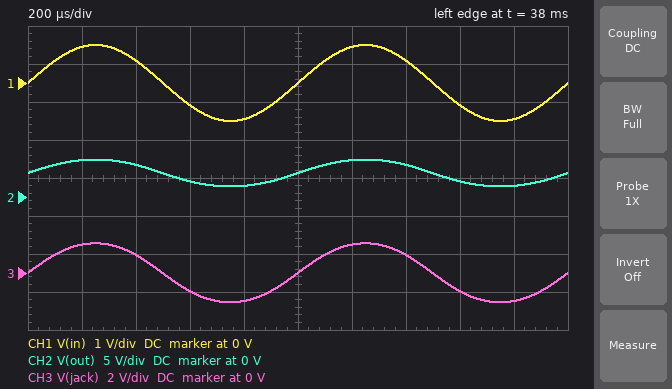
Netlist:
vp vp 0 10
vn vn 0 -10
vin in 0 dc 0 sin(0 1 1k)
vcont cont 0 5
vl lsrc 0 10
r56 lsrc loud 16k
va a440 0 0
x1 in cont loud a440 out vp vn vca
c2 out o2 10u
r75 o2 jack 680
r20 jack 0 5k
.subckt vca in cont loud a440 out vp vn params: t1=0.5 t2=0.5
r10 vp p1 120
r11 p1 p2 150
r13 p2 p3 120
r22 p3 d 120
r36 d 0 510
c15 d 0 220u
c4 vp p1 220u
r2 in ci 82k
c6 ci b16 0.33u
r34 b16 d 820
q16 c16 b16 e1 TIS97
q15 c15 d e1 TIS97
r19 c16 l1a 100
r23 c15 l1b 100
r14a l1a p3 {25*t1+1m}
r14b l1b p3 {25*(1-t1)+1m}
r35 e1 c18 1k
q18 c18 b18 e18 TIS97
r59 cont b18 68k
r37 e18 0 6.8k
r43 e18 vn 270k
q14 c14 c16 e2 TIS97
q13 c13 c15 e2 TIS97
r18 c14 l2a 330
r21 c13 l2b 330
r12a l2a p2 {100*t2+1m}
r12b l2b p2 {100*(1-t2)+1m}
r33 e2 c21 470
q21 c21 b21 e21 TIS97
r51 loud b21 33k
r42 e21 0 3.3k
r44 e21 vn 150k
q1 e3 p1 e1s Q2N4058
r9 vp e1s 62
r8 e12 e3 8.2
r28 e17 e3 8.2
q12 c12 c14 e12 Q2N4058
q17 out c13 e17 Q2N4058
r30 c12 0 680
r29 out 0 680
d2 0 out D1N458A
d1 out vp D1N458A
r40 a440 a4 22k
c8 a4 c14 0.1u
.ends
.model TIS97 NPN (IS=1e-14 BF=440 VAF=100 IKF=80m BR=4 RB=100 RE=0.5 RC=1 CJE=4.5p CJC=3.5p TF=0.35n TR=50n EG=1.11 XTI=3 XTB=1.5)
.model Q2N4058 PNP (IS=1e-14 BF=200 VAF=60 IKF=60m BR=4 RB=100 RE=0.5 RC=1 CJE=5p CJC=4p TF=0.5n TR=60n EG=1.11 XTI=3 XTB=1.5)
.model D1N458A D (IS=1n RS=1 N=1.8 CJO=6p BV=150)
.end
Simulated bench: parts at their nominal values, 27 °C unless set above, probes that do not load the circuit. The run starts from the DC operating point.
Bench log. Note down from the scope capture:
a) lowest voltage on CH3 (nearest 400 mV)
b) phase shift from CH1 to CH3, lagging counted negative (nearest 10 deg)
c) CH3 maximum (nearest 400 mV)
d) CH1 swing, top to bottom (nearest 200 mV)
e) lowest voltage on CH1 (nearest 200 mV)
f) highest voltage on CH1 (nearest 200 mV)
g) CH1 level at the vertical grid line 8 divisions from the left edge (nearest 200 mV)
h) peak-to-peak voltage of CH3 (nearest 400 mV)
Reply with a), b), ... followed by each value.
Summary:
a) -1.6 V
b) 0 deg
c) 1.6 V
d) 2.0 V
e) -1.0 V
f) 1.0 V
g) -600 mV
h) 3.2 V
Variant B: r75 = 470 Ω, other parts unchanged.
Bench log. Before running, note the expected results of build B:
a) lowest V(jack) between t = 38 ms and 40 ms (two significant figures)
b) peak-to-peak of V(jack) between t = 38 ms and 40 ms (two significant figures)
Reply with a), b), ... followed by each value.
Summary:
a) -1.6 V
b) 3.2 V
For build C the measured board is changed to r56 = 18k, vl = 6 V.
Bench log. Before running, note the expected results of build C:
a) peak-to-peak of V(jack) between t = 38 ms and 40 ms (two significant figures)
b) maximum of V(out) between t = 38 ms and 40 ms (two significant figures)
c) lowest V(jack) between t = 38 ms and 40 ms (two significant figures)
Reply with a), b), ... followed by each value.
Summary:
a) 3.2 V
b) 5.0 V
c) -1.6 V
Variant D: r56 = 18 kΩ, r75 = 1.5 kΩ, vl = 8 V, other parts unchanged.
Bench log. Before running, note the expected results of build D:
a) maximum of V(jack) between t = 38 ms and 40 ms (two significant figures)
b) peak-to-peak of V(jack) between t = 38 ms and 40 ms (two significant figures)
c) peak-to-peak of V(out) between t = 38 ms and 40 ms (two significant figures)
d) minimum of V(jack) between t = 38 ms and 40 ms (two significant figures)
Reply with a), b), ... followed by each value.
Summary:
a) 1.4 V
b) 2.8 V
c) 3.6 V
d) -1.4 V
